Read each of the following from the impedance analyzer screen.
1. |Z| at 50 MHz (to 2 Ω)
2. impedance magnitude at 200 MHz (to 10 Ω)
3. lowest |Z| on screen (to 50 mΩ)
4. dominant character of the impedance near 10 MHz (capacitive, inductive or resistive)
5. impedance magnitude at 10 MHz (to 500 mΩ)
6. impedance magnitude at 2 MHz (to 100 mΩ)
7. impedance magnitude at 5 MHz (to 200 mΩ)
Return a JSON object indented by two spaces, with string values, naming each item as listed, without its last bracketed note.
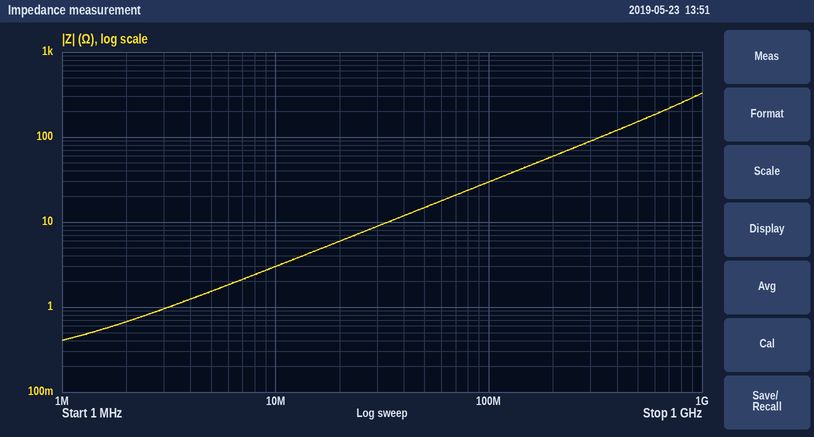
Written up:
{
  "|Z| at 50 MHz": "14 Ω",
  "impedance magnitude at 200 MHz": "60 Ω",
  "lowest |Z| on screen": "400 mΩ",
  "dominant character of the impedance near 10 MHz": "inductive",
  "impedance magnitude at 10 MHz": "3.0 Ω",
  "impedance magnitude at 2 MHz": "700 mΩ",
  "impedance magnitude at 5 MHz": "1.6 Ω"
}
